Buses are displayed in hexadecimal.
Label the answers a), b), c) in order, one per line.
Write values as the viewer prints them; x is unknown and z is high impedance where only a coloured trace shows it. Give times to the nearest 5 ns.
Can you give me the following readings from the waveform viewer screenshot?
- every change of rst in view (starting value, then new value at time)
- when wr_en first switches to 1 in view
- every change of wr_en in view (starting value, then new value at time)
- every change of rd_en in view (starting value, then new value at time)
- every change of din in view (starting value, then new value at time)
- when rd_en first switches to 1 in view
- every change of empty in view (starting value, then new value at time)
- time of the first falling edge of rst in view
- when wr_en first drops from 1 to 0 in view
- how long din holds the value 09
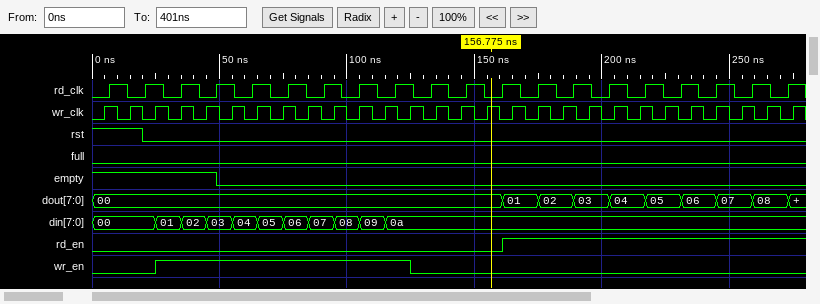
a) 1, 0 at 20 ns
b) 25 ns
c) 0, 1 at 25 ns, 0 at 125 ns
d) 0, 1 at 160 ns
e) 00, 01 at 25 ns, 02 at 35 ns, 03 at 45 ns, 04 at 55 ns, 05 at 65 ns, 06 at 75 ns, 07 at 85 ns, 08 at 95 ns, 09 at 105 ns, 0a at 115 ns
f) 160 ns
g) 1, 0 at 50 ns
h) 20 ns
i) 125 ns
j) 10 ns
